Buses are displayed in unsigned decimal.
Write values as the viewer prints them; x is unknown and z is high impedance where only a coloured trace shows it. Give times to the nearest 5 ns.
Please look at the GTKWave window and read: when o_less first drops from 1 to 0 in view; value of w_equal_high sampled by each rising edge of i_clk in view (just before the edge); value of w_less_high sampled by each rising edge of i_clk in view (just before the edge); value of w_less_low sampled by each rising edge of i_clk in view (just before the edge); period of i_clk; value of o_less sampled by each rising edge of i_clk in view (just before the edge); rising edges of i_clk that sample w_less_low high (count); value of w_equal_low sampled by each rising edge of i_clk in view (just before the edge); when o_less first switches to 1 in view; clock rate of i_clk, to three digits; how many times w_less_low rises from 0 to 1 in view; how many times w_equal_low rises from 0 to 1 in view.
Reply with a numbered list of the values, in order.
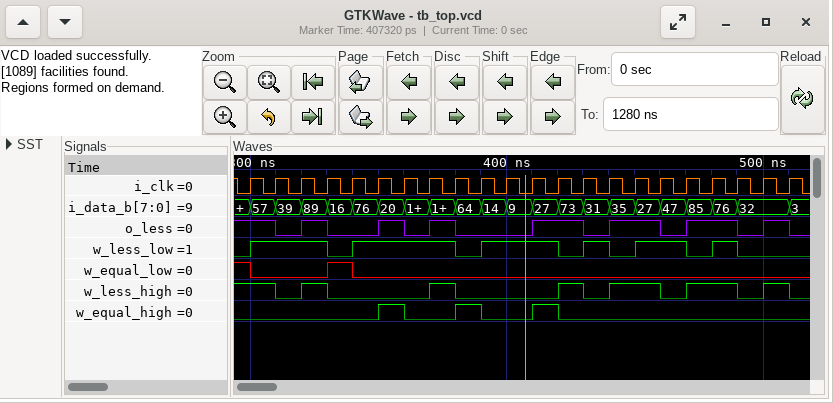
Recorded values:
1. 310 ns
2. 0 0 0 0 0 0 1 0 0 1 0 0 1 0 0 0 0 0 0 0 0 0
3. 1 1 0 1 0 0 0 0 1 0 0 0 0 1 0 1 1 0 1 1 0 1
4. 0 1 1 1 0 1 1 1 1 0 1 1 1 0 1 0 1 1 0 1 0 0
5. 10 ns
6. 1 1 0 1 0 0 1 0 1 0 0 0 1 1 0 1 1 0 1 1 0 1
7. 14
8. 1 0 0 0 1 0 0 0 0 0 0 0 0 0 0 0 0 0 0 0 0 0
9. 320 ns
10. 100 MHz
11. 6
12. 1
